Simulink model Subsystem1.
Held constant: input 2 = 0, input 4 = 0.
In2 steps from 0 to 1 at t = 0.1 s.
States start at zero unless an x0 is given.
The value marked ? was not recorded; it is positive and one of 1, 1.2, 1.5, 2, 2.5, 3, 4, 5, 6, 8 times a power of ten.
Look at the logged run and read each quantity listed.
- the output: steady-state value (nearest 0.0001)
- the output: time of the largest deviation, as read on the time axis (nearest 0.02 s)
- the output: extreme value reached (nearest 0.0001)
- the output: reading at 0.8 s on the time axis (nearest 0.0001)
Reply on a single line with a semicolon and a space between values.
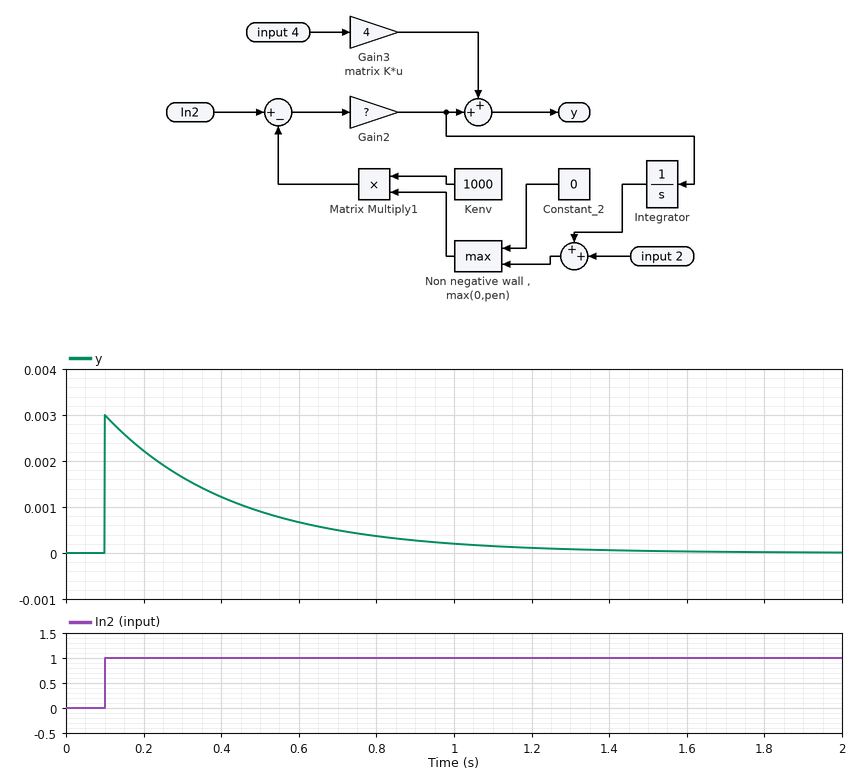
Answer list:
0.0000; 0.10 s; 0.0030; 0.0004
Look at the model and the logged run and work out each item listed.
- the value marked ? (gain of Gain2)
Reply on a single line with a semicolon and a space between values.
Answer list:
0.003
